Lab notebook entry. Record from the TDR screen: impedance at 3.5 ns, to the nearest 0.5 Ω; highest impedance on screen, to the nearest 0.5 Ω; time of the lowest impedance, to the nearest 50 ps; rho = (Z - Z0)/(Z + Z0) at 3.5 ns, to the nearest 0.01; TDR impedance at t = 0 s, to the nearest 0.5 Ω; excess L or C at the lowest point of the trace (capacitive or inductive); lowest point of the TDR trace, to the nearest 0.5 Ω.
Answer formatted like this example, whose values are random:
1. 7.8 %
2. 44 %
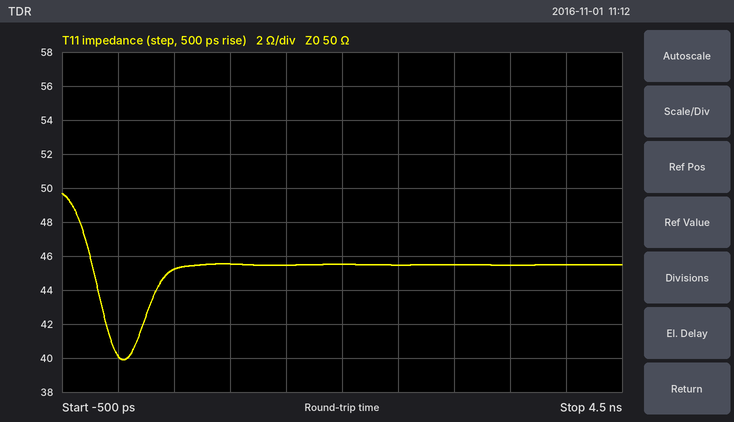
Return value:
1. 45.5 Ω
2. 49.5 Ω
3. 50 ps
4. -0.05
5. 40.0 Ω
6. capacitive
7. 40.0 Ω
